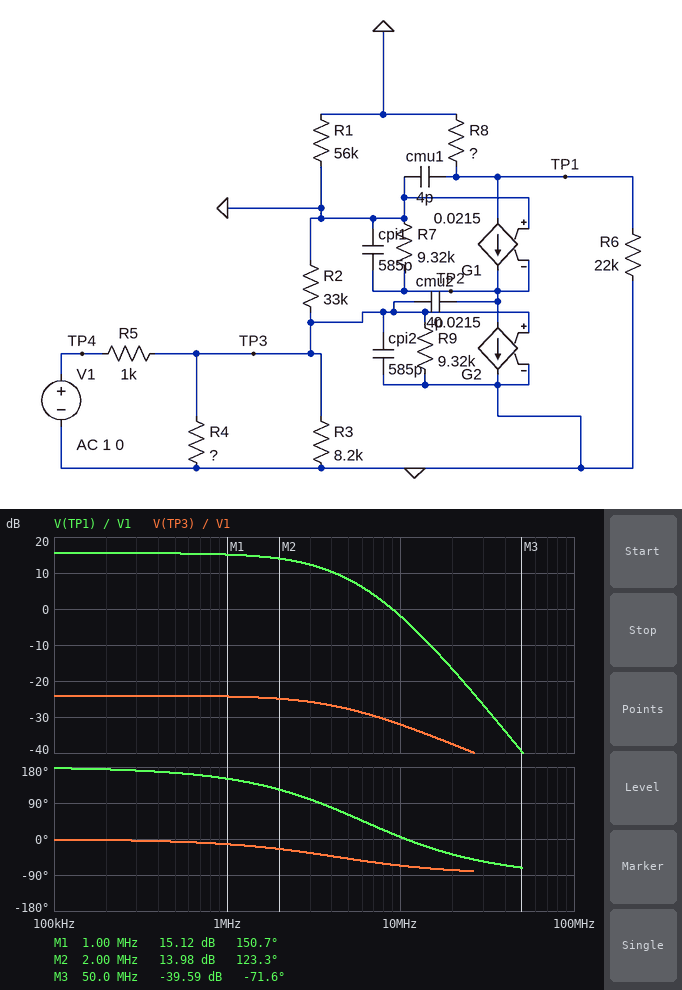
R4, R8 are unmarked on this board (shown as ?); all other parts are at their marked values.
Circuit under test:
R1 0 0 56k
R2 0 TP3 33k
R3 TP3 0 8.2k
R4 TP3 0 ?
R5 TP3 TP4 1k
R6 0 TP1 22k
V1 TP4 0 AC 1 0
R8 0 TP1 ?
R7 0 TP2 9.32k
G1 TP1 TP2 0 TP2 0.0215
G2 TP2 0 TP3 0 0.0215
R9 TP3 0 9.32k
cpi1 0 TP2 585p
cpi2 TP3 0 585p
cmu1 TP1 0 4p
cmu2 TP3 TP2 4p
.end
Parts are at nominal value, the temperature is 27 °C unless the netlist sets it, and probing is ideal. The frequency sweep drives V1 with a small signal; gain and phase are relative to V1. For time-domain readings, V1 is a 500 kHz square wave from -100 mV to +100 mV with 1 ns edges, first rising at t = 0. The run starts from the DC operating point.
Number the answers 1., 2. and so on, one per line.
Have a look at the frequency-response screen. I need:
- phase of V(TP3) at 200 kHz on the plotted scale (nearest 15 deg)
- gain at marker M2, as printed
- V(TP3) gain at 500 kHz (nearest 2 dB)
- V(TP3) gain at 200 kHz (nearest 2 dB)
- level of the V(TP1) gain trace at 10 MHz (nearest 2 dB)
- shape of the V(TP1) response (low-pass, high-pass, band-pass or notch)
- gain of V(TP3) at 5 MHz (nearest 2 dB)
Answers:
1. 0 deg
2. 13.98 dB
3. -24 dB
4. -24 dB
5. -2 dB
6. low-pass
7. -28 dB
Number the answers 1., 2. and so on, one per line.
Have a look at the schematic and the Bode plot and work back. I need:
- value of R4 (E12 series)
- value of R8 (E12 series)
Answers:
1. 68 Ω
2. 5.6 kΩ
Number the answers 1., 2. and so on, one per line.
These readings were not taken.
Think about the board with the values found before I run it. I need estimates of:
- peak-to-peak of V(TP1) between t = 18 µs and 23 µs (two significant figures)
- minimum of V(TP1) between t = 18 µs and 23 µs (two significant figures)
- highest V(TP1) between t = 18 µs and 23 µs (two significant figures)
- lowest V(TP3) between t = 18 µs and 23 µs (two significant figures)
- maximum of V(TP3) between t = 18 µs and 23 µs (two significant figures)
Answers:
1. 1.2 V
2. -600 mV
3. 600 mV
4. -6.3 mV
5. 6.3 mV
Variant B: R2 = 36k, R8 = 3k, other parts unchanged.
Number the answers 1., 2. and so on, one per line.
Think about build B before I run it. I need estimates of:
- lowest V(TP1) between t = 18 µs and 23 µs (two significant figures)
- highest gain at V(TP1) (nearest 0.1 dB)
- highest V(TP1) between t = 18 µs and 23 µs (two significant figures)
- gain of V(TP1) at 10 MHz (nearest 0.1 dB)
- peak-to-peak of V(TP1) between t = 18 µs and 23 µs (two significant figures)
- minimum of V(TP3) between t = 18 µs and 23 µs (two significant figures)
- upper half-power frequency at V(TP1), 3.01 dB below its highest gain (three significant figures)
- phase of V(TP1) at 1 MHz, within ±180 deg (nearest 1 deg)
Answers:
1. -350 mV
2. 11.0 dB
3. 350 mV
4. -4.6 dB
5. 710 mV
6. -6.3 mV
7. 3.05 MHz
8. 153 deg
